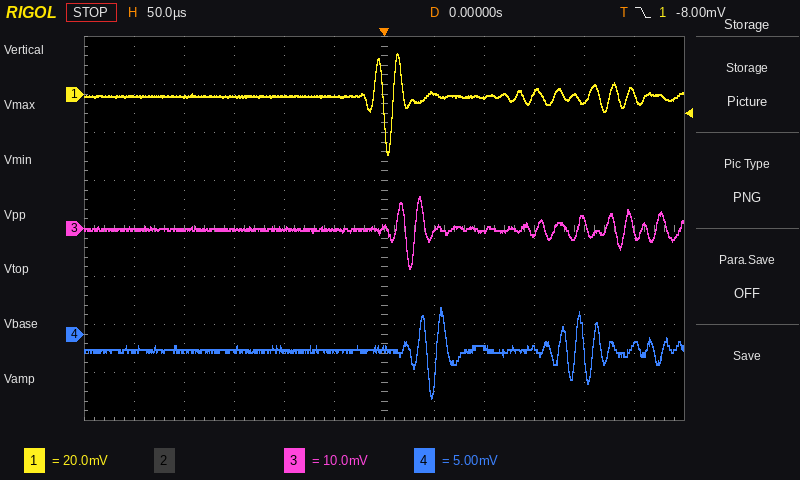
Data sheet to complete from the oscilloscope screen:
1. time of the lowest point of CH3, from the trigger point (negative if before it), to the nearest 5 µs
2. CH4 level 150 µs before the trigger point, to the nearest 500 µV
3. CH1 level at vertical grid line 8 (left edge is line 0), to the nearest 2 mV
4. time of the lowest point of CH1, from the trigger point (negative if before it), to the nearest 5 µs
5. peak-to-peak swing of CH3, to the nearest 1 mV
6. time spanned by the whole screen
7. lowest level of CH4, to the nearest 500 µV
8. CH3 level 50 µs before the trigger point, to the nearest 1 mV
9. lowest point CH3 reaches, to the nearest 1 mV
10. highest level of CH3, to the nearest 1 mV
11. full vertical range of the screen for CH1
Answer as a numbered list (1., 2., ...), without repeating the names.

1. +25 µs
2. -1.5 mV
3. -2 mV
4. +5 µs
5. 15 mV
6. 600 µs
7. -6.5 mV
8. 0 mV
9. -8 mV
10. 7 mV
11. 160 mV
